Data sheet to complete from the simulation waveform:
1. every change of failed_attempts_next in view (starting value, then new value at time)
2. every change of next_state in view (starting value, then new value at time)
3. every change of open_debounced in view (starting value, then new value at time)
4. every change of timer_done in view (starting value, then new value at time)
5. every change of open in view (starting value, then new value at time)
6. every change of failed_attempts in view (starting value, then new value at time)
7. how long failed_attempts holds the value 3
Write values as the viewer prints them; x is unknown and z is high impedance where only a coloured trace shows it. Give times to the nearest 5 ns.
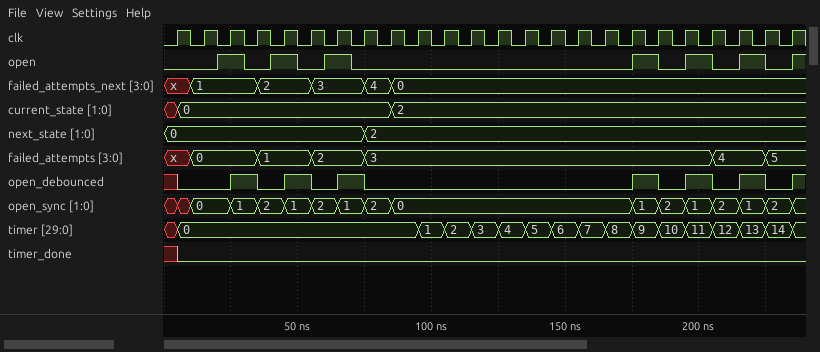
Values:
x, 1 at 10 ns, 2 at 35 ns, 3 at 55 ns, 4 at 75 ns, 0 at 85 ns
0, 2 at 75 ns
x, 0 at 5 ns, 1 at 25 ns, 0 at 35 ns, 1 at 45 ns, 0 at 55 ns, 1 at 65 ns, 0 at 75 ns, 1 at 175 ns, 0 at 185 ns, 1 at 195 ns, 0 at 205 ns, 1 at 215 ns, 0 at 225 ns, 1 at 235 ns
x, 0 at 5 ns
0, 1 at 20 ns, 0 at 30 ns, 1 at 40 ns, 0 at 50 ns, 1 at 60 ns, 0 at 70 ns, 1 at 175 ns, 0 at 185 ns, 1 at 195 ns, 0 at 205 ns, 1 at 215 ns, 0 at 225 ns, 1 at 235 ns
x, 0 at 10 ns, 1 at 35 ns, 2 at 55 ns, 3 at 75 ns, 4 at 205 ns, 5 at 225 ns
130 ns
